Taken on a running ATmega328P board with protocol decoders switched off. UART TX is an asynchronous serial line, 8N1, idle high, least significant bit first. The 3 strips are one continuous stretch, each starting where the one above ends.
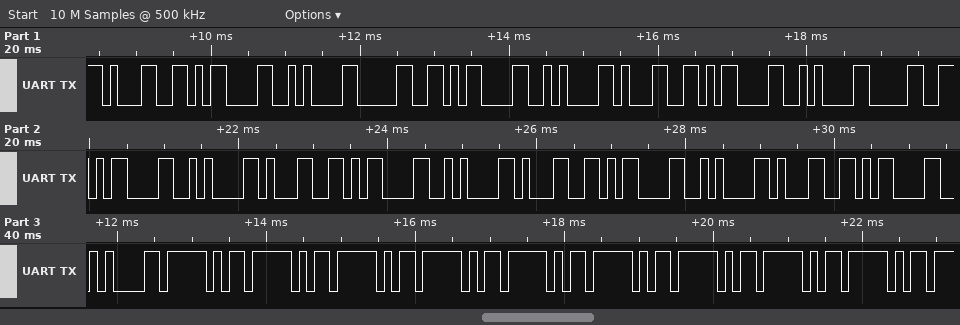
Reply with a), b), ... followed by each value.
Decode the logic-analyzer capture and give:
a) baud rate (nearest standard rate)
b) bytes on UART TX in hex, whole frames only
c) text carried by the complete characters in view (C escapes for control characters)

a) 9600 baud
b) 31 0D 0A 30 0D 0A 31 0D 0A 30 0D 0A 31 0D 0A 31 0D 0A 31 0D 0A 5F 5F 5F 5F 5F 5F 5F 5F 5F
c) "1\r\n0\r\n1\r\n0\r\n1\r\n1\r\n1\r\n_________"
